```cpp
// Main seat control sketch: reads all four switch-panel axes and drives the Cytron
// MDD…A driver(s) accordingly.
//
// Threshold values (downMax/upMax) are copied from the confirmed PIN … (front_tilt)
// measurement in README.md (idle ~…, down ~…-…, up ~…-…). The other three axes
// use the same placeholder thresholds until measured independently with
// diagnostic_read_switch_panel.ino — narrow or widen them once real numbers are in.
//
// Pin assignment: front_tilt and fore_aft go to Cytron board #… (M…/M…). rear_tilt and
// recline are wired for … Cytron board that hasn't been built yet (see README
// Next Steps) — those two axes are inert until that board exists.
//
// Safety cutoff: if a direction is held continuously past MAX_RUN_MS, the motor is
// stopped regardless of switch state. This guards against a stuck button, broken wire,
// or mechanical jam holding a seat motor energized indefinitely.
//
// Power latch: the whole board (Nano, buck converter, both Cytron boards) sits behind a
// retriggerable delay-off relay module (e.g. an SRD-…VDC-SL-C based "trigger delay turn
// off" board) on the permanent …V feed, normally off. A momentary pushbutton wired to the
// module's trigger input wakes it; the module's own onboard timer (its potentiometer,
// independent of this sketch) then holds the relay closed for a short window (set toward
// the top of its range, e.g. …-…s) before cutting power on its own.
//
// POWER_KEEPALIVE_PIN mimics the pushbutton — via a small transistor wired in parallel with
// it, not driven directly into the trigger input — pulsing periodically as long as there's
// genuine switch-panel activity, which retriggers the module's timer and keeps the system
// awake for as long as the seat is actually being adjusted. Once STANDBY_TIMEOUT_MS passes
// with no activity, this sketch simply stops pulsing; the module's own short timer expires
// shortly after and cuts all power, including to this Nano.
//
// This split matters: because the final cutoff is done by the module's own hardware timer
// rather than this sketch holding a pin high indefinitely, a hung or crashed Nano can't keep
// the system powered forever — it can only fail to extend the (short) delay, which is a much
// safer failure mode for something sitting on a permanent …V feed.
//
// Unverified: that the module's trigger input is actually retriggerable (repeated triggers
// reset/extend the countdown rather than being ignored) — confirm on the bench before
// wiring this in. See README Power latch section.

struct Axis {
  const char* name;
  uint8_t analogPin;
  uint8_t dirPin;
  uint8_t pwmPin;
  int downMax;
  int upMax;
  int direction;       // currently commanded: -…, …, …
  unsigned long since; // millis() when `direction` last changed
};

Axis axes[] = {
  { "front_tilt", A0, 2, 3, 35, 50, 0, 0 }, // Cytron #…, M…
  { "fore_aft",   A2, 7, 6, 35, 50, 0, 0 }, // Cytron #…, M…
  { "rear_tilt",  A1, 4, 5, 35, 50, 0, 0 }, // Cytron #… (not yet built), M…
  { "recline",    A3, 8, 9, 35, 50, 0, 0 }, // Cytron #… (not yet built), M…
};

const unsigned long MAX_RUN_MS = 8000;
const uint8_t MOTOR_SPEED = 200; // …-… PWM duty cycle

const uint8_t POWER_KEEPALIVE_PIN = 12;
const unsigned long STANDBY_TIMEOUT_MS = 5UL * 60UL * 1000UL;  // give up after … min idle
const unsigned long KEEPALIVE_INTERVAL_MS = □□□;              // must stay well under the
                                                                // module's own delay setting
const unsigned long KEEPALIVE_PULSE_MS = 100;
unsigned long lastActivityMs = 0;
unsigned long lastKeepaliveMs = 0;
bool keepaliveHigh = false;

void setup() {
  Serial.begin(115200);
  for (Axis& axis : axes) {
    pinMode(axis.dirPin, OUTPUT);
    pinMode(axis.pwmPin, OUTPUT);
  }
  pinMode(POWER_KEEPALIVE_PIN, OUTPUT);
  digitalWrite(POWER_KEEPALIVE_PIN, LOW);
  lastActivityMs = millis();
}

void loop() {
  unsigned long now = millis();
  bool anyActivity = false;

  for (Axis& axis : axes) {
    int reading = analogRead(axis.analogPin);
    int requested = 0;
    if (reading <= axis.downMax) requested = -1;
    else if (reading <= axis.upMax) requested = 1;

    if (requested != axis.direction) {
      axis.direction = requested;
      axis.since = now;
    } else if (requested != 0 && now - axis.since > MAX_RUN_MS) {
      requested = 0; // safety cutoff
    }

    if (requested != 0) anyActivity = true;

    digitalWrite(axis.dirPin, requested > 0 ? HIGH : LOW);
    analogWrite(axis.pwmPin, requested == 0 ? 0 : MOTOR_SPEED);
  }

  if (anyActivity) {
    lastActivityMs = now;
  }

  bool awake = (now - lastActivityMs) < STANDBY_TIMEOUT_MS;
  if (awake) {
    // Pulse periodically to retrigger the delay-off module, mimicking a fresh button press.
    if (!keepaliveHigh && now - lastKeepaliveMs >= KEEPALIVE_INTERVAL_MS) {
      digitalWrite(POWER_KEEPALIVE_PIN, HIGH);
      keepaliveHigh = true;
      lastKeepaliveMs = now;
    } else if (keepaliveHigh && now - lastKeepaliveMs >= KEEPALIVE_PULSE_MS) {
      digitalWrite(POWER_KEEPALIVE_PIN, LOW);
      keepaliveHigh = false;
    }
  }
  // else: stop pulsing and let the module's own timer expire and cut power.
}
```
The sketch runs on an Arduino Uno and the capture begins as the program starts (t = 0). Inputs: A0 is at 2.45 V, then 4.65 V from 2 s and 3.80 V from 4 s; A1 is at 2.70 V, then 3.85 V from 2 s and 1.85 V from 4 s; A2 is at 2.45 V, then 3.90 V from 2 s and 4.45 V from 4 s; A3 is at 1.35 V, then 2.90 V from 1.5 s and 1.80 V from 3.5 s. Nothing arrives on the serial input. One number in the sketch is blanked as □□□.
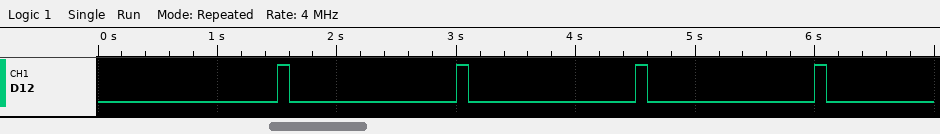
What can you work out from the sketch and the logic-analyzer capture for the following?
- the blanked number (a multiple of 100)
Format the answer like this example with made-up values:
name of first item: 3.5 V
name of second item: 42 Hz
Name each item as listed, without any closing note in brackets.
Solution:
the blanked number: 1500
